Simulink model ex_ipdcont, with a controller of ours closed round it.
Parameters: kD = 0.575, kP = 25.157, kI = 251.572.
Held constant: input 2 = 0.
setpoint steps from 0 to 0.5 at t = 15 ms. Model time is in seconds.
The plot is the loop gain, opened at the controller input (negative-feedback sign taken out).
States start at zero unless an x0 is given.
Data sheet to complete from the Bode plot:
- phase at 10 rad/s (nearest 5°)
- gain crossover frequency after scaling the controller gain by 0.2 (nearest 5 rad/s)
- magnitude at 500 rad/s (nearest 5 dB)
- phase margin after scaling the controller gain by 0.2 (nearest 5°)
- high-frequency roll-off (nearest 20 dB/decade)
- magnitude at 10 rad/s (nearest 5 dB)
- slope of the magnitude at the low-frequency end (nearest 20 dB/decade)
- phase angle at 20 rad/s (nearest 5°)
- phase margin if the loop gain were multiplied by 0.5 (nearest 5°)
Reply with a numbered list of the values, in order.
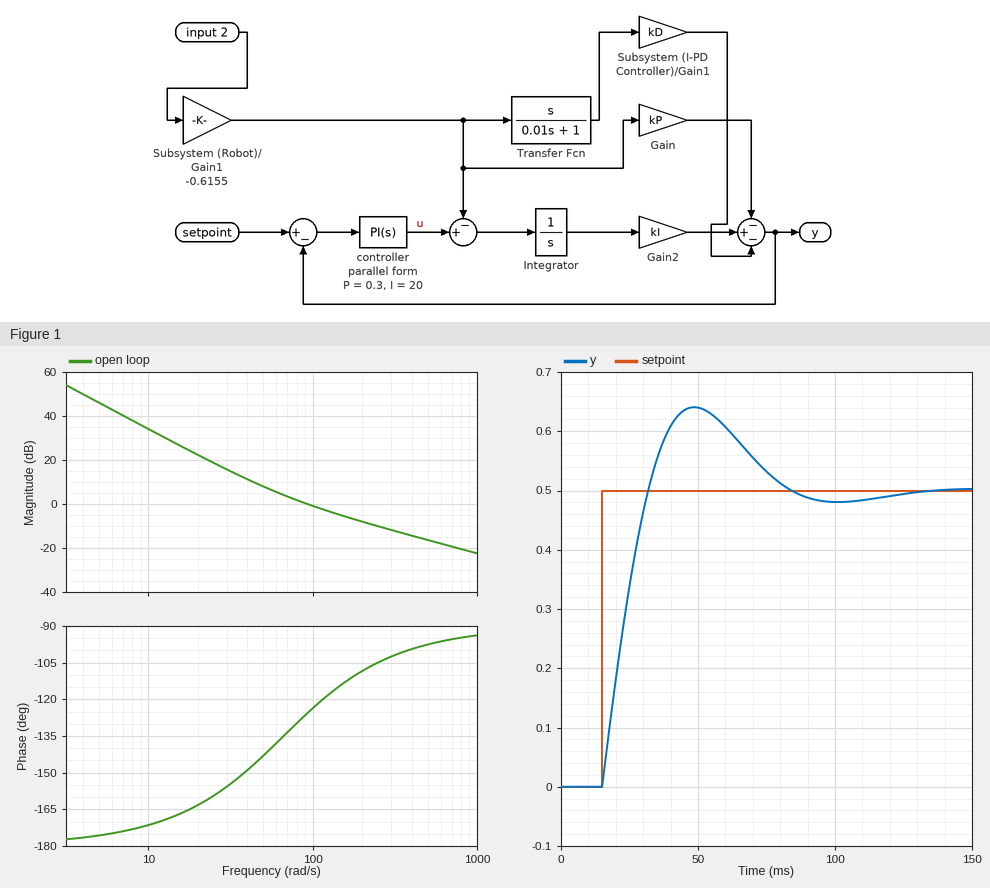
1. -170°
2. 35 rad/s
3. -15 dB
4. 25°
5. -20 dB/decade
6. 35 dB
7. -40 dB/decade
8. -165°
9. 40°
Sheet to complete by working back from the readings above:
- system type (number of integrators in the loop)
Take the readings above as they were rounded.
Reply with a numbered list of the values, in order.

1. 2
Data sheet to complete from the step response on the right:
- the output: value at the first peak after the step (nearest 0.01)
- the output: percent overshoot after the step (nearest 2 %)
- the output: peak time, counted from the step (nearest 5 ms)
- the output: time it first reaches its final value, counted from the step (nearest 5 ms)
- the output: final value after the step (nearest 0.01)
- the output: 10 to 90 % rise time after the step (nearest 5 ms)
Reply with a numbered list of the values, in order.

1. 0.64
2. 28 %
3. 35 ms
4. 15 ms
5. 0.50
6. 15 ms
